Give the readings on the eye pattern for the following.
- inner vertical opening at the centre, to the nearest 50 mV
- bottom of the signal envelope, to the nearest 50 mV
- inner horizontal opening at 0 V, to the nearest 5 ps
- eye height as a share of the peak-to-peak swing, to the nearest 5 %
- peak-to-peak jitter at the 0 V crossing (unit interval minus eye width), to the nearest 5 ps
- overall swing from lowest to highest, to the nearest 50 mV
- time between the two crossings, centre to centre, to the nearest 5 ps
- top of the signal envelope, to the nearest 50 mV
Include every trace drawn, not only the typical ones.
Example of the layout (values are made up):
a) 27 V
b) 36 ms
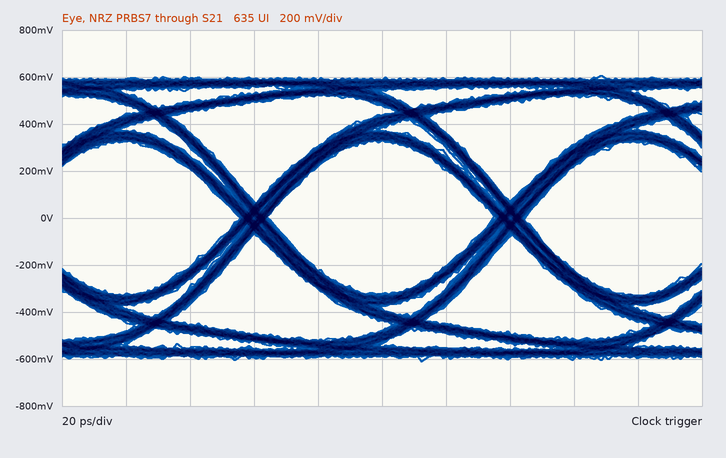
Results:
a) 650 mV
b) -600 mV
c) 70 ps
d) 55 %
e) 10 ps
f) 1.20 V
g) 80 ps
h) 600 mV
